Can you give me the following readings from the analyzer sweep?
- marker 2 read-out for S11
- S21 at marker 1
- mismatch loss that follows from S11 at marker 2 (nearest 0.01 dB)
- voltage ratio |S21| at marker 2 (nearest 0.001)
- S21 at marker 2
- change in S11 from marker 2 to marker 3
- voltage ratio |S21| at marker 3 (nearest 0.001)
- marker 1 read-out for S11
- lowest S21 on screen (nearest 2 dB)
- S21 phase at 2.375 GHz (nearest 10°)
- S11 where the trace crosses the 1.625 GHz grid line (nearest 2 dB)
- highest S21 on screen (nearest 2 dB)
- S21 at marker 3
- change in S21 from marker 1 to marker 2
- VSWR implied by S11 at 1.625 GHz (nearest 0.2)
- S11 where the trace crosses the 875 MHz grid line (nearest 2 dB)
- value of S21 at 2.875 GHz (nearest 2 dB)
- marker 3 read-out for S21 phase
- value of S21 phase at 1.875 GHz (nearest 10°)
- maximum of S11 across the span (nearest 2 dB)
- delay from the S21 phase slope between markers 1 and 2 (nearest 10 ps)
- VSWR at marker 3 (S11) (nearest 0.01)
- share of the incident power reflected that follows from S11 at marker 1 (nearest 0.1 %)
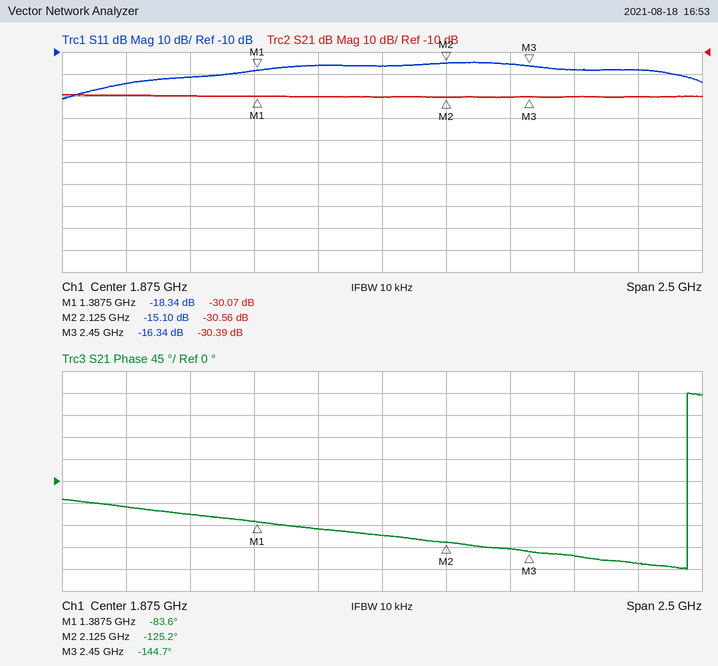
-15.10 dB
-30.07 dB
0.14 dB
0.030
-30.56 dB
-1.24 dB
0.030
-18.34 dB
-30 dB
-140°
-16 dB
-30 dB
-30.39 dB
-0.49 dB
1.4
-24 dB
-30 dB
-144.7°
-110°
-14 dB
160 ps
1.36
1.5 %
